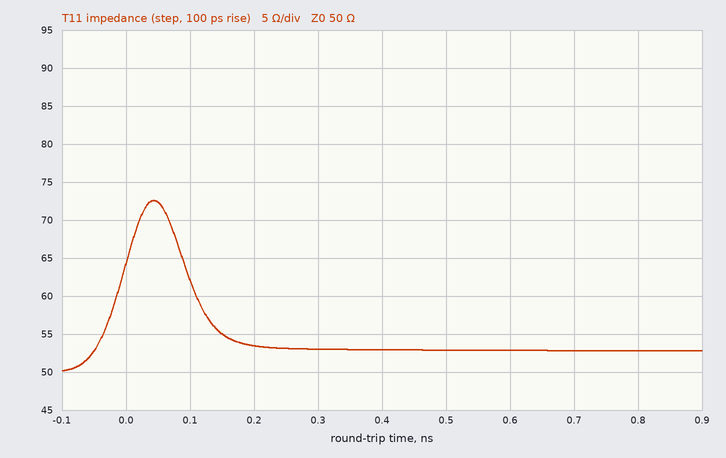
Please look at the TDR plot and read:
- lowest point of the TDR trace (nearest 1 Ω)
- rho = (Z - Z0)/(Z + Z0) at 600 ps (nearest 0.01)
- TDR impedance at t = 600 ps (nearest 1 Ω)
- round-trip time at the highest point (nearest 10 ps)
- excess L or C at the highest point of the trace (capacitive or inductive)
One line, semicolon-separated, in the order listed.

50 Ω; +0.03; 53 Ω; 40 ps; inductive
